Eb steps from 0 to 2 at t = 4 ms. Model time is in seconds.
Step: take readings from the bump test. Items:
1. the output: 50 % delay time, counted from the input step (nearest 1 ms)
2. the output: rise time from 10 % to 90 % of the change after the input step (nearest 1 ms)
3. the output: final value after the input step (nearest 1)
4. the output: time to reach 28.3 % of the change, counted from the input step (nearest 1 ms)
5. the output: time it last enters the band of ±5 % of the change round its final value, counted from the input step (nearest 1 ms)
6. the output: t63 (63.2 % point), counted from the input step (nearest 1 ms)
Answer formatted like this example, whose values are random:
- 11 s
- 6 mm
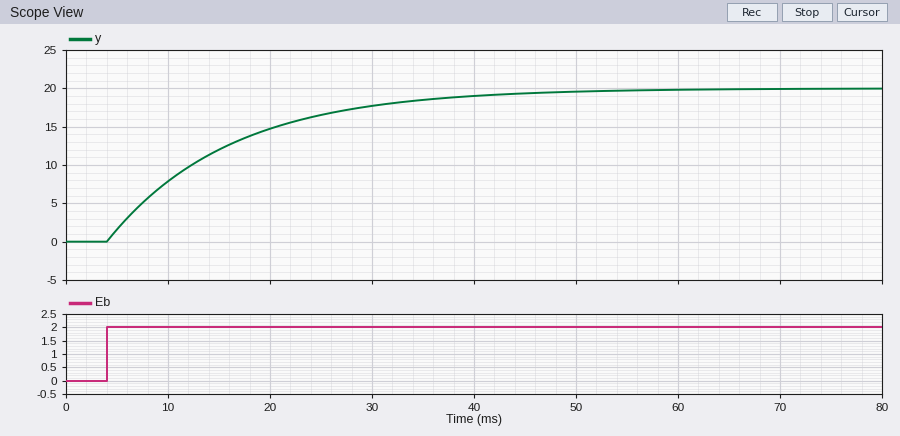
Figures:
- 8 ms
- 26 ms
- 20
- 4 ms
- 36 ms
- 12 ms
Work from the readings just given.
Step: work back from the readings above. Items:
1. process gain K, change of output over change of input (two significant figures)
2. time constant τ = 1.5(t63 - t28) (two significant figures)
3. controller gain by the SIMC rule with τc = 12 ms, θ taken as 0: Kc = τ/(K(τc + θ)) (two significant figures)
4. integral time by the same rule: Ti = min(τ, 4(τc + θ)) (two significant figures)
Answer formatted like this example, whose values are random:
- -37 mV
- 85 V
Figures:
- 10
- 12 ms
- 0.10
- 12 ms
